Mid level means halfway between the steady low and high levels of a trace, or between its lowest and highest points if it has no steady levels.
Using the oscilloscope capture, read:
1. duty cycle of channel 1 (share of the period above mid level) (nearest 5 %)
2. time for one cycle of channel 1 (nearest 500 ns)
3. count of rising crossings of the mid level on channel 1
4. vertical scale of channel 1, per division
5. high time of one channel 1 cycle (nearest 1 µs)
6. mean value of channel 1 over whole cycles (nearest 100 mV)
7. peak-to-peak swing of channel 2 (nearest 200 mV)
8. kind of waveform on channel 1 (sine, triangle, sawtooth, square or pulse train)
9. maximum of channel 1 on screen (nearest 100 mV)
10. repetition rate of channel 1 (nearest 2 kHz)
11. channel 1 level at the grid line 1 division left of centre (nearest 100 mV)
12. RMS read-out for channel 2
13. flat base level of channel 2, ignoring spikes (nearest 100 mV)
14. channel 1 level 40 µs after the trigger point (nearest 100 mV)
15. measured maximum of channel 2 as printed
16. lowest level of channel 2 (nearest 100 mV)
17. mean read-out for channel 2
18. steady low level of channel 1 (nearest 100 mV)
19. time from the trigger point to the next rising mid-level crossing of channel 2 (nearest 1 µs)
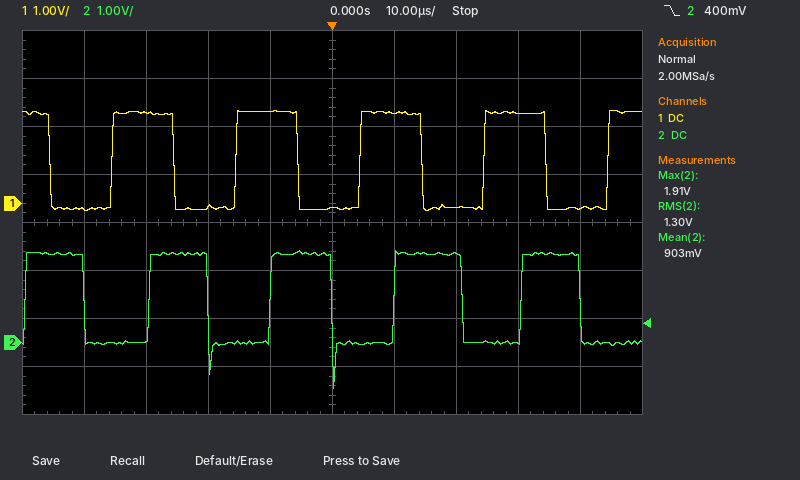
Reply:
50 %
20.0 µs
5
1 V
10 µs
900 mV
2.8 V
square
1.9 V
50 kHz
1.9 V
1.30 V
0.0 V
-100 mV
1.91 V
-1.0 V
903 mV
-100 mV
10 µs
